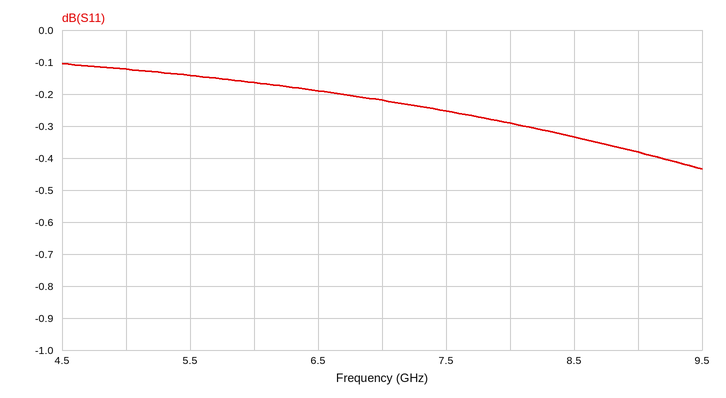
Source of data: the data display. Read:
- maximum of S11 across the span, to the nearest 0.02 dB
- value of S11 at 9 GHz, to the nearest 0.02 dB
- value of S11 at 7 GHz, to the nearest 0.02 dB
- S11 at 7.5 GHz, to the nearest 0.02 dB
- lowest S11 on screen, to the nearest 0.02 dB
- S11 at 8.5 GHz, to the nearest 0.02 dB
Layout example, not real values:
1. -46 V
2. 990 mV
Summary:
1. -0.10 dB
2. -0.38 dB
3. -0.22 dB
4. -0.26 dB
5. -0.44 dB
6. -0.34 dB
